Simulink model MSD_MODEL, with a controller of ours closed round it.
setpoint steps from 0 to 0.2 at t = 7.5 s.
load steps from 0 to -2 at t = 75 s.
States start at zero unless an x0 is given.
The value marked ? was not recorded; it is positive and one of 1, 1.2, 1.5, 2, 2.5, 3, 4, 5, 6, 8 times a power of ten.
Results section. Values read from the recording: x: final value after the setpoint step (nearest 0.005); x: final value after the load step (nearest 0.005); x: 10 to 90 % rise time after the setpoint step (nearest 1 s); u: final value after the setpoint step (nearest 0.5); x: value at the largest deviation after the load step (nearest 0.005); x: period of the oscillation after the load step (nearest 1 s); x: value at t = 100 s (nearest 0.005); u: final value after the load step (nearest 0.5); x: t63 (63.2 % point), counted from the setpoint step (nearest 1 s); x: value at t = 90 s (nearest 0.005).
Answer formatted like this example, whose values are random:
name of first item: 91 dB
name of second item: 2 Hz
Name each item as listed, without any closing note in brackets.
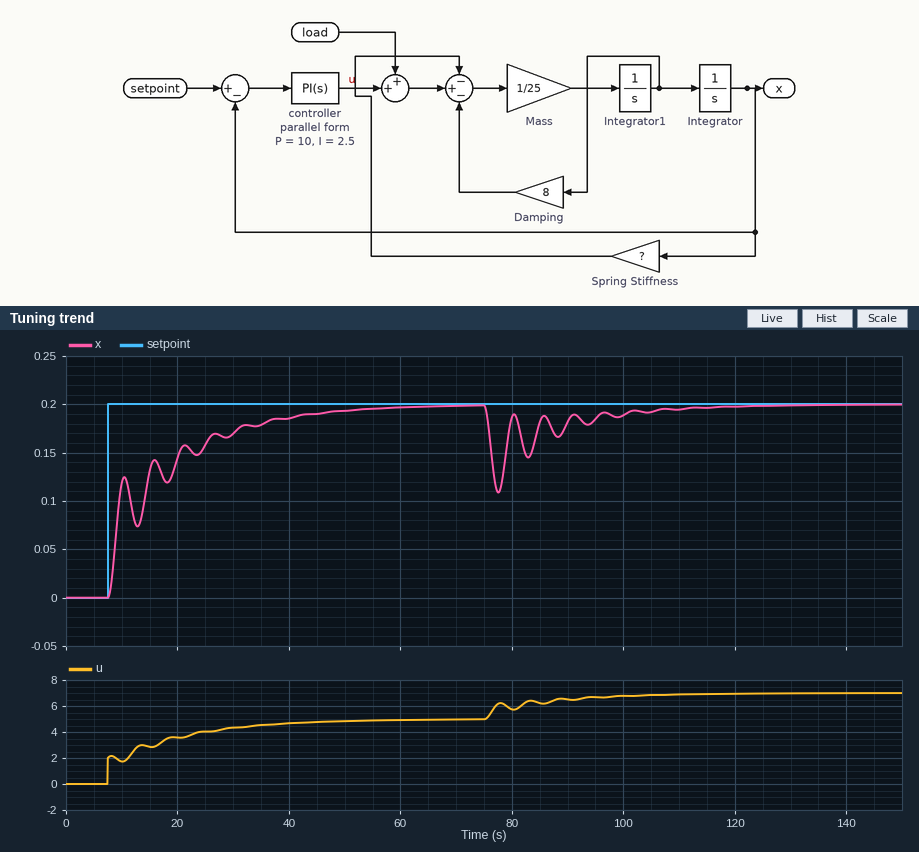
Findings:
x: final value after the setpoint step: 0.200
x: final value after the load step: 0.200
x: 10 to 90 % rise time after the setpoint step: 27 s
u: final value after the setpoint step: 5.0
x: value at the largest deviation after the load step: 0.110
x: period of the oscillation after the load step: 5 s
x: value at t = 100 s: 0.190
u: final value after the load step: 7.0
x: t63 (63.2 % point), counted from the setpoint step: 7 s
x: value at t = 90 s: 0.180
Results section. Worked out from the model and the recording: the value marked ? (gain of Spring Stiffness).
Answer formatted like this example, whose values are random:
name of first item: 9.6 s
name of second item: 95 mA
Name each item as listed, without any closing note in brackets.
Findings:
the value marked ?: 25
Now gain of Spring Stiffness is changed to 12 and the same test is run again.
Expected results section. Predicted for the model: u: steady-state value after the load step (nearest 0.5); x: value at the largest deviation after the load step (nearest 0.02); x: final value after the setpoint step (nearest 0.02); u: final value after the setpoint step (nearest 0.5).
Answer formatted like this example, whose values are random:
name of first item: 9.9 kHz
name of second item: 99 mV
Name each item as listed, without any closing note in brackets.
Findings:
u: steady-state value after the load step: 4.5
x: value at the largest deviation after the load step: 0.06
x: final value after the setpoint step: 0.20
u: final value after the setpoint step: 2.5
